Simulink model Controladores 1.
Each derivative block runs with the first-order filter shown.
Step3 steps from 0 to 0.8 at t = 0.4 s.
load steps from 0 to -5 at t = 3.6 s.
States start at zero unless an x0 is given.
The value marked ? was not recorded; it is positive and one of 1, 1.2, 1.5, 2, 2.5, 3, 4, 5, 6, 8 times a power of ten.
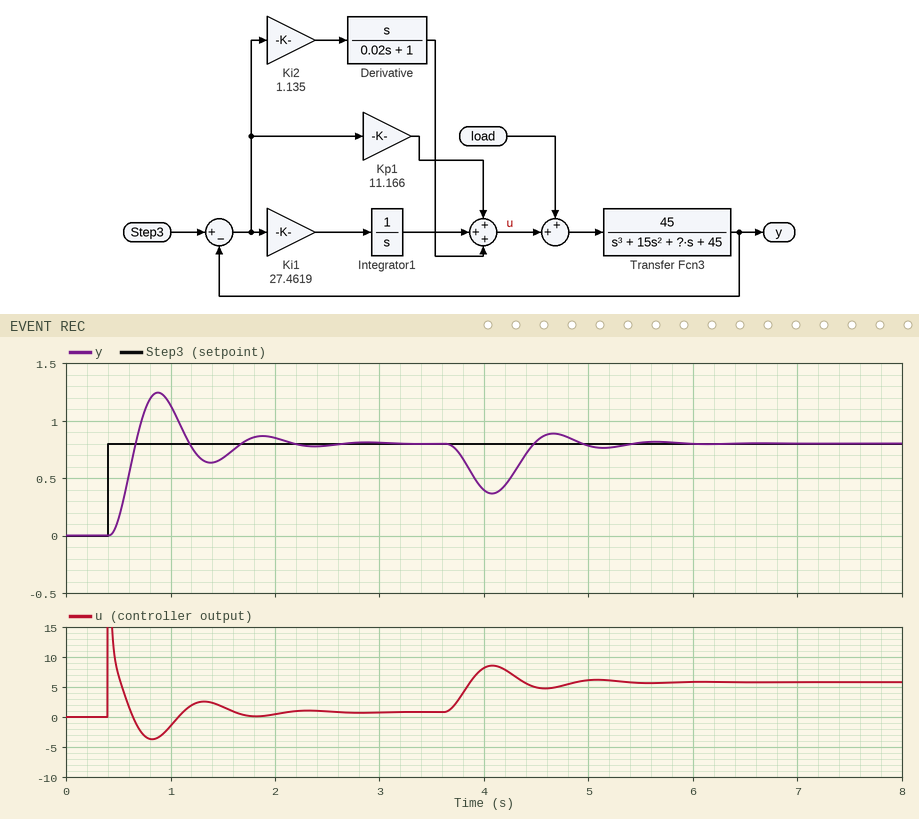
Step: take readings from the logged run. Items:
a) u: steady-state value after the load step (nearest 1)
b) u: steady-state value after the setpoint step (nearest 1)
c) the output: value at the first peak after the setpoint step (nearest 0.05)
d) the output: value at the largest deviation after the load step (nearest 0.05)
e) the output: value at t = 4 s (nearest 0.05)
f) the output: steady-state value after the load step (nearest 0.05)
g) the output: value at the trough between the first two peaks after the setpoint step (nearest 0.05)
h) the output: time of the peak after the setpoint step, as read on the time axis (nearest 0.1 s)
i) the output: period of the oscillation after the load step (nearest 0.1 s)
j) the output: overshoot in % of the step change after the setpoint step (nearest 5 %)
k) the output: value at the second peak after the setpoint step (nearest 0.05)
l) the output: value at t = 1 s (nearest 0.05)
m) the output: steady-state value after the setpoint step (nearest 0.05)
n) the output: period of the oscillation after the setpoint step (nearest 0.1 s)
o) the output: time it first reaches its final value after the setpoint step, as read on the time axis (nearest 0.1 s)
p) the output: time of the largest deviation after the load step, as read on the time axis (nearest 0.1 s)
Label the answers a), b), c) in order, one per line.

a) 6
b) 1
c) 1.25
d) 0.35
e) 0.40
f) 0.80
g) 0.65
h) 0.9 s
i) 1.1 s
j) 55 %
k) 0.85
l) 1.15
m) 0.80
n) 1.0 s
o) 0.7 s
p) 4.1 s
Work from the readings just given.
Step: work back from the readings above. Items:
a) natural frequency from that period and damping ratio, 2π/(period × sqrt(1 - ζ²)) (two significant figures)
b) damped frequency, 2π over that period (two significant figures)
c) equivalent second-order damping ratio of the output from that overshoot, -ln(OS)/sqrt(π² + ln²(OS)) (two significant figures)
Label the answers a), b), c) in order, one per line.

a) 6.4 rad/s
b) 6.3 rad/s
c) 0.19
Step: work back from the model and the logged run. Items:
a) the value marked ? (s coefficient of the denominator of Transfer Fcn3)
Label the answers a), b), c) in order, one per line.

a) 60
